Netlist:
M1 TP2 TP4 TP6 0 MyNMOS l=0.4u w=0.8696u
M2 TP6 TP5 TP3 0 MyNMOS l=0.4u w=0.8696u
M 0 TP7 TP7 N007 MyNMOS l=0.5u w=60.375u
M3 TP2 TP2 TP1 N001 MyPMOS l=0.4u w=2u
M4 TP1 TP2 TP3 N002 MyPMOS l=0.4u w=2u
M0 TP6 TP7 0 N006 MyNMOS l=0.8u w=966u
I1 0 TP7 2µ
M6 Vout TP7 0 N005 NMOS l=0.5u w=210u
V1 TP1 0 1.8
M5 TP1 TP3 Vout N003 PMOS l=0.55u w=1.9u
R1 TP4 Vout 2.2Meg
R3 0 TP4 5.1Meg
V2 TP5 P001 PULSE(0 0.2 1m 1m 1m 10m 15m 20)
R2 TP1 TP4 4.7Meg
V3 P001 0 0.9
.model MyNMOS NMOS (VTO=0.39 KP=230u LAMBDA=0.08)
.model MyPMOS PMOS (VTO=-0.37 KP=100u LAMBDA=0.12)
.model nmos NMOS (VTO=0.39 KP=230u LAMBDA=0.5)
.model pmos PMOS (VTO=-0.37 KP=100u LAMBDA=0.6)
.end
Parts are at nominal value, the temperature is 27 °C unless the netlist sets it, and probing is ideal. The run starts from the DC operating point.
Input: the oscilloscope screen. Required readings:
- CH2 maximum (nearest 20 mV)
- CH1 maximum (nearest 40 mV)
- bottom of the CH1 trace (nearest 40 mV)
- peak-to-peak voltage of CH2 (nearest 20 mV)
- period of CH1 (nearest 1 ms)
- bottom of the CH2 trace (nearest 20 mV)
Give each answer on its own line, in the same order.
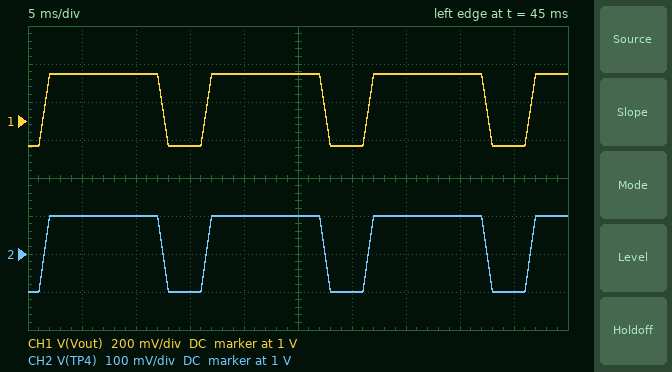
1.10 V
1.24 V
880 mV
200 mV
15 ms
900 mV
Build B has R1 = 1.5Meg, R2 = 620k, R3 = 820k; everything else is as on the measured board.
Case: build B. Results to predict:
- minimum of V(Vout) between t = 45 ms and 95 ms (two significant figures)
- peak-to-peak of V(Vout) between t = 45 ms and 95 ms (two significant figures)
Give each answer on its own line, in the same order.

370 mV
1.0 V
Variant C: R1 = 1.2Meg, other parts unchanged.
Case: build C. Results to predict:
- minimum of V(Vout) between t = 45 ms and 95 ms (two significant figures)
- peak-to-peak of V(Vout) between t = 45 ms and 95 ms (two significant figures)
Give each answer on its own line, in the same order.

880 mV
300 mV
